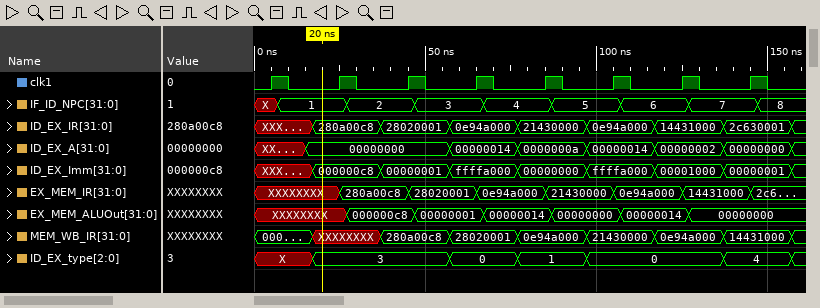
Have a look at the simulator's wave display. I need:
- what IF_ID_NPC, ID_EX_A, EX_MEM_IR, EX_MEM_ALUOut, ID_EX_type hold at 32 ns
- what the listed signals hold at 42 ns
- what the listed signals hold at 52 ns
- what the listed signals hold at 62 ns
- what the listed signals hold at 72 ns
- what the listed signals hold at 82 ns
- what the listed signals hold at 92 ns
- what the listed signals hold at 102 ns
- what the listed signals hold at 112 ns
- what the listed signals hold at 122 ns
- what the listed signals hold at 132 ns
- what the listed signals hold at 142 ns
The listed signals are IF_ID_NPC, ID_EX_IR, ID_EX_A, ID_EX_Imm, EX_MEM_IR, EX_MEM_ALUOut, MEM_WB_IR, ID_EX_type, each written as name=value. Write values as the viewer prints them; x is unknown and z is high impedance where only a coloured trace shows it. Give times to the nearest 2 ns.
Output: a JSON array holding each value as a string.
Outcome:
["IF_ID_NPC=2, ID_EX_A=00000000, EX_MEM_IR=280a00c8, EX_MEM_ALUOut=000000c8, ID_EX_type=3", "IF_ID_NPC=2, ID_EX_IR=28020001, ID_EX_A=00000000, ID_EX_Imm=00000001, EX_MEM_IR=280a00c8, EX_MEM_ALUOut=000000c8, MEM_WB_IR=280a00c8, ID_EX_type=3", "IF_ID_NPC=3, ID_EX_IR=28020001, ID_EX_A=00000000, ID_EX_Imm=00000001, EX_MEM_IR=28020001, EX_MEM_ALUOut=00000001, MEM_WB_IR=280a00c8, ID_EX_type=3", "IF_ID_NPC=3, ID_EX_IR=0e94a000, ID_EX_A=00000014, ID_EX_Imm=ffffa000, EX_MEM_IR=28020001, EX_MEM_ALUOut=00000001, MEM_WB_IR=28020001, ID_EX_type=0", "IF_ID_NPC=4, ID_EX_IR=0e94a000, ID_EX_A=00000014, ID_EX_Imm=ffffa000, EX_MEM_IR=0e94a000, EX_MEM_ALUOut=00000014, MEM_WB_IR=28020001, ID_EX_type=0", "IF_ID_NPC=4, ID_EX_IR=21430000, ID_EX_A=0000000a, ID_EX_Imm=00000000, EX_MEM_IR=0e94a000, EX_MEM_ALUOut=00000014, MEM_WB_IR=0e94a000, ID_EX_type=1", "IF_ID_NPC=5, ID_EX_IR=21430000, ID_EX_A=0000000a, ID_EX_Imm=00000000, EX_MEM_IR=21430000, EX_MEM_ALUOut=00000000, MEM_WB_IR=0e94a000, ID_EX_type=1", "IF_ID_NPC=5, ID_EX_IR=0e94a000, ID_EX_A=00000014, ID_EX_Imm=ffffa000, EX_MEM_IR=21430000, EX_MEM_ALUOut=00000000, MEM_WB_IR=21430000, ID_EX_type=0", "IF_ID_NPC=6, ID_EX_IR=0e94a000, ID_EX_A=00000014, ID_EX_Imm=ffffa000, EX_MEM_IR=0e94a000, EX_MEM_ALUOut=00000014, MEM_WB_IR=21430000, ID_EX_type=0", "IF_ID_NPC=6, ID_EX_IR=14431000, ID_EX_A=00000002, ID_EX_Imm=00001000, EX_MEM_IR=0e94a000, EX_MEM_ALUOut=00000014, MEM_WB_IR=0e94a000, ID_EX_type=0", "IF_ID_NPC=7, ID_EX_IR=14431000, ID_EX_A=00000002, ID_EX_Imm=00001000, EX_MEM_IR=14431000, EX_MEM_ALUOut=00000000, MEM_WB_IR=0e94a000, ID_EX_type=0", "IF_ID_NPC=7, ID_EX_IR=2c630001, ID_EX_A=00000000, ID_EX_Imm=00000001, EX_MEM_IR=14431000, EX_MEM_ALUOut=00000000, MEM_WB_IR=14431000, ID_EX_type=4"]
